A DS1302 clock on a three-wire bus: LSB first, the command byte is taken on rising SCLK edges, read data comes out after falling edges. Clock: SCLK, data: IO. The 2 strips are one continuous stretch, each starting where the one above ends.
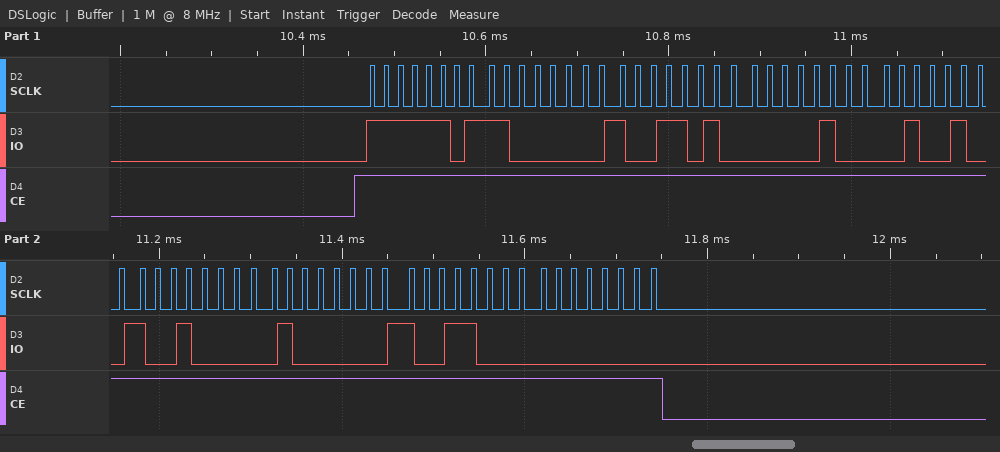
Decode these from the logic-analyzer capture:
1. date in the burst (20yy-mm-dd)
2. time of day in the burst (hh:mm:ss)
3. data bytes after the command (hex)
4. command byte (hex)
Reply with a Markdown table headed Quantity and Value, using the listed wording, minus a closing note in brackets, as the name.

| Quantity | Value |
|---|---|
| date in the burst | 2019-09-24 |
| time of day in the burst | 20:59:03 |
| data bytes after the command | 03 59 20 24 09 02 19 00 |
| command byte | 0xBF |
